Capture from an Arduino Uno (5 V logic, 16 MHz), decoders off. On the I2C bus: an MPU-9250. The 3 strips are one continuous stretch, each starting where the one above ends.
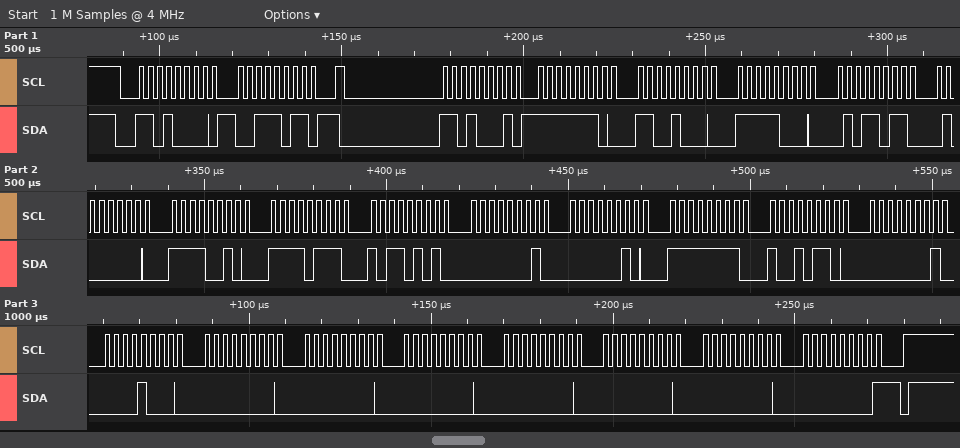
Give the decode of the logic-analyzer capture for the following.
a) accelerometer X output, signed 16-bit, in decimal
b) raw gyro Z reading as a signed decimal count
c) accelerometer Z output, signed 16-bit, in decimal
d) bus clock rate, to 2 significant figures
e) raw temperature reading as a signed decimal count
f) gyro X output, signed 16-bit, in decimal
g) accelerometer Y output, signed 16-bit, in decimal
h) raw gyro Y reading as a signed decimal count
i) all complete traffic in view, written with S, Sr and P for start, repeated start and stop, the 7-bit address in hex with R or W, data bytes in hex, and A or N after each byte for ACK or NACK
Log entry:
-312
264
16626
400 kHz
-2123
258
-1957
-106
S 68W A 3B A Sr 68R A FE A C8 A F8 A 5B A 40 A F2 A F7 A B5 A 01 A 02 A FF A 96 A 01 A 08 A 00 A 00 A 00 A 00 A 00 A 00 A 00 N P
